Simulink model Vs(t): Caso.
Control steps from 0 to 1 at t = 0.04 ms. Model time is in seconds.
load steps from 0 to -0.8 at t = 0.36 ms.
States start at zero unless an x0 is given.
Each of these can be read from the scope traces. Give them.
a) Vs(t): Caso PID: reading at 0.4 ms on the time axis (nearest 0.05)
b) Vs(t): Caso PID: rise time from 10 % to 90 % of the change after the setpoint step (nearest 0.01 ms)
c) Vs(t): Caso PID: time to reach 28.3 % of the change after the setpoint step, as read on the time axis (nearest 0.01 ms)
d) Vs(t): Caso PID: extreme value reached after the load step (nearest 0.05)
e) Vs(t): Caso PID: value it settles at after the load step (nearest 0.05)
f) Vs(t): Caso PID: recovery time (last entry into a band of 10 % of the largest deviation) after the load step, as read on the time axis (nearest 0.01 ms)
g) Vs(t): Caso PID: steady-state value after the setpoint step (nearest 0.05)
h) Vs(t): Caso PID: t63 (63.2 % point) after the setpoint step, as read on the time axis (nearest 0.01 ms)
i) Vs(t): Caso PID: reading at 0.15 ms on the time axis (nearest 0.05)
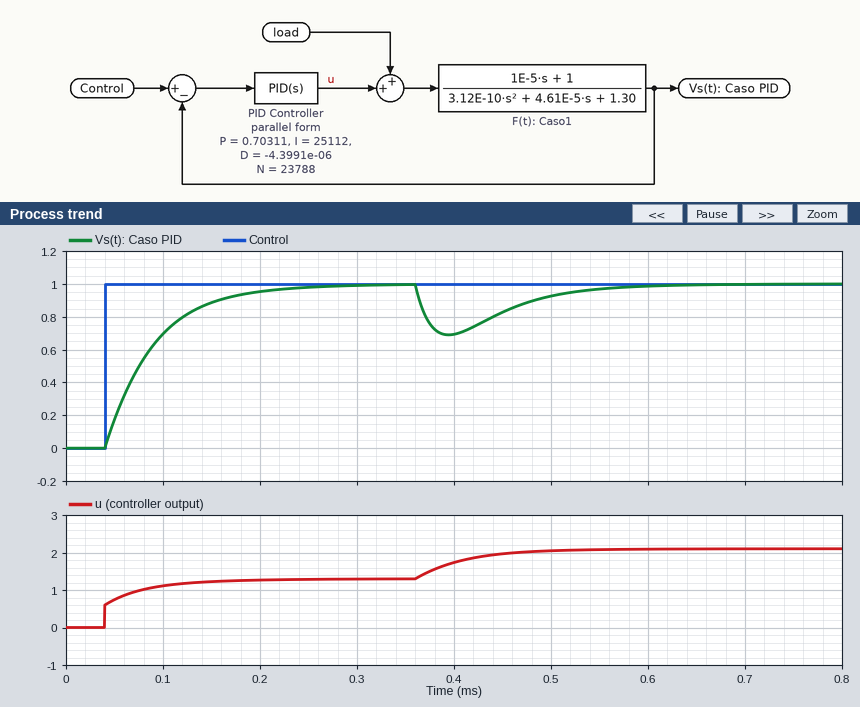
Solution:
0.70
0.11 ms
0.06 ms
0.70
1.00
0.55 ms
1.00
0.09 ms
0.90
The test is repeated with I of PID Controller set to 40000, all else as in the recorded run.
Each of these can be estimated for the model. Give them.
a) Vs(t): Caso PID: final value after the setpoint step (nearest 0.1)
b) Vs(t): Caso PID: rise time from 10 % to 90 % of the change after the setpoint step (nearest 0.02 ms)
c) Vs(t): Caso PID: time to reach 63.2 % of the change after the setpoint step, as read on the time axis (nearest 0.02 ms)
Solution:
1.0
0.06 ms
0.08 ms
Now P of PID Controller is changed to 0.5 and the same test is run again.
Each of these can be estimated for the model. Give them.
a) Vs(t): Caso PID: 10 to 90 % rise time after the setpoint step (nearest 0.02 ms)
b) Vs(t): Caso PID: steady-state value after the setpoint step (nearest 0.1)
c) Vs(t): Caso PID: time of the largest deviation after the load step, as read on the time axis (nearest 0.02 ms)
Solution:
0.10 ms
1.0
0.40 ms
